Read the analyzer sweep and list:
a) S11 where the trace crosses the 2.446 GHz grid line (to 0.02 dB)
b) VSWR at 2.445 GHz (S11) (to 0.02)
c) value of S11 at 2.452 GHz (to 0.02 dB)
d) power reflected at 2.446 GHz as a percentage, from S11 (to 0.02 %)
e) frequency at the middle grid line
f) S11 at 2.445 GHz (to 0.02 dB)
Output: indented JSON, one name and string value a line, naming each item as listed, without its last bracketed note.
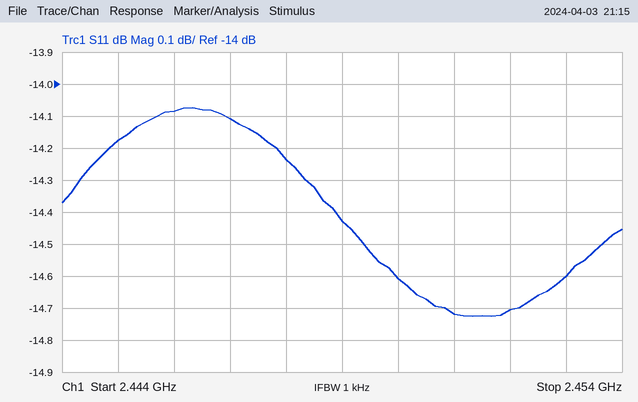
{
  "S11 where the trace crosses the 2.446 GHz grid line": "-14.08 dB",
  "VSWR at 2.445 GHz (S11)": "1.48",
  "value of S11 at 2.452 GHz": "-14.70 dB",
  "power reflected at 2.446 GHz as a percentage, from S11": "3.90 %",
  "frequency at the middle grid line": "2.449 GHz",
  "S11 at 2.445 GHz": "-14.18 dB"
}
